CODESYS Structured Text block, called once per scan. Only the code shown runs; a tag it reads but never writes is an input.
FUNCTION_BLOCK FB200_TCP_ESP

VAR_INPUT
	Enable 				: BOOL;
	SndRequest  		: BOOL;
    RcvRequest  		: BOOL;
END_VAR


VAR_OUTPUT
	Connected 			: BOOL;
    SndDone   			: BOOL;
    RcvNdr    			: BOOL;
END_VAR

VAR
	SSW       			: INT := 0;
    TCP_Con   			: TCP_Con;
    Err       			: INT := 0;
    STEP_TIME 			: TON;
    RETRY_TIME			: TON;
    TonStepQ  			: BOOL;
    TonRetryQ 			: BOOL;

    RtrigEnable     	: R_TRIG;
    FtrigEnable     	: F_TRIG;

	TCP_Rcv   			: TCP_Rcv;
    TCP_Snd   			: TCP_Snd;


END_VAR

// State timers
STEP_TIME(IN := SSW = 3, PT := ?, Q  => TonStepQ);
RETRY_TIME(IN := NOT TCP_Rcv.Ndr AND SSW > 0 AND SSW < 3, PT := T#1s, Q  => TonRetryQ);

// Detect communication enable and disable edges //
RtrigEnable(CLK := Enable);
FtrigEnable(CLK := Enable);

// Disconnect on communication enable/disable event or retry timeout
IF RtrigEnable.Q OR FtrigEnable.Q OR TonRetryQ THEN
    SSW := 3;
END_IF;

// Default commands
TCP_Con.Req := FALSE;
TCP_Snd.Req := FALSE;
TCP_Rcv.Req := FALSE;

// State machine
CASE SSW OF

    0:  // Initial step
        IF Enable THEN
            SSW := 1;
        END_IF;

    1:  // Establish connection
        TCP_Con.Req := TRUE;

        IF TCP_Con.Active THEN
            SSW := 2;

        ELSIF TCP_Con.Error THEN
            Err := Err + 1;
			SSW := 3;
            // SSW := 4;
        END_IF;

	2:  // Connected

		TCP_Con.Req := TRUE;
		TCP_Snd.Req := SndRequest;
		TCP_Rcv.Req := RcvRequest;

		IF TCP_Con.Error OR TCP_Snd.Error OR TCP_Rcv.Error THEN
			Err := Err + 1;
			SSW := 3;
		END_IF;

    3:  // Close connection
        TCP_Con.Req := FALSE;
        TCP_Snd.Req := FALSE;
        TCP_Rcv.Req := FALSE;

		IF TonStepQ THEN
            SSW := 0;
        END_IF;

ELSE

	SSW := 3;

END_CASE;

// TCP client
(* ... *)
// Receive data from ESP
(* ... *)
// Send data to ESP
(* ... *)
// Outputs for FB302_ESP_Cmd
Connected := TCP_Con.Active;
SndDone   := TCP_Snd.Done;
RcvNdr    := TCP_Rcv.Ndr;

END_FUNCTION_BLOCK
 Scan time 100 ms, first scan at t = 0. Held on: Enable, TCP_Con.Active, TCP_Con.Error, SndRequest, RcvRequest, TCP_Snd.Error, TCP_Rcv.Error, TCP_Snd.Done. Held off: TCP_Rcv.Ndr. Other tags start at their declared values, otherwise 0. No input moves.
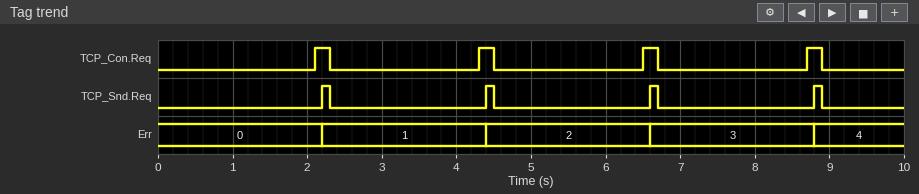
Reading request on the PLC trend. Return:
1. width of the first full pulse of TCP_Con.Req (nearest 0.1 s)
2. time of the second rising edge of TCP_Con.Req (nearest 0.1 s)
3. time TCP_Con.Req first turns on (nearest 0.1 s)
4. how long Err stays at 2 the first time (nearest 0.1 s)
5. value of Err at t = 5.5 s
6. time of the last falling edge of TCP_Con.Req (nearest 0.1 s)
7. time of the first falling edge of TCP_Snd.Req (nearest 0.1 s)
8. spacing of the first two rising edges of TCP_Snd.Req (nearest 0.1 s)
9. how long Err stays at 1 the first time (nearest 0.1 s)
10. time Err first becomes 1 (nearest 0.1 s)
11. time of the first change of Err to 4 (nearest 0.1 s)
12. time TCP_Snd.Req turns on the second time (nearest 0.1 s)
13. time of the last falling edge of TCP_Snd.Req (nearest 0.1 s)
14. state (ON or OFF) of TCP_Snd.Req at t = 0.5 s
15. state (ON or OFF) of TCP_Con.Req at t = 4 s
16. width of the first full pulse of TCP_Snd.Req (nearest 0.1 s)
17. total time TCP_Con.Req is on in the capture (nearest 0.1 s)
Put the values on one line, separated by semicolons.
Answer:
0.2 s; 4.3 s; 2.1 s; 2.2 s; 2; 8.9 s; 2.3 s; 2.2 s; 2.2 s; 2.2 s; 8.8 s; 4.4 s; 8.9 s; OFF; OFF; 0.1 s; 0.8 s
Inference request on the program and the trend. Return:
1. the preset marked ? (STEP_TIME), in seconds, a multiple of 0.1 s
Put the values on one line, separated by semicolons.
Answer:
1.8 s
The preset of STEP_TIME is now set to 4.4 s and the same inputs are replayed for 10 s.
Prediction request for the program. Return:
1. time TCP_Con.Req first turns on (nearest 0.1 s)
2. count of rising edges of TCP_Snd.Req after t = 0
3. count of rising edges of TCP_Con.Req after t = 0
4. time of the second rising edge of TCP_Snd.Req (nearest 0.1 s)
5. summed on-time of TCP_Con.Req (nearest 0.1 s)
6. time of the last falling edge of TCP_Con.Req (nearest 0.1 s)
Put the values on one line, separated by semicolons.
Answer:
4.7 s; 2; 2; 9.6 s; 0.4 s; 9.7 s
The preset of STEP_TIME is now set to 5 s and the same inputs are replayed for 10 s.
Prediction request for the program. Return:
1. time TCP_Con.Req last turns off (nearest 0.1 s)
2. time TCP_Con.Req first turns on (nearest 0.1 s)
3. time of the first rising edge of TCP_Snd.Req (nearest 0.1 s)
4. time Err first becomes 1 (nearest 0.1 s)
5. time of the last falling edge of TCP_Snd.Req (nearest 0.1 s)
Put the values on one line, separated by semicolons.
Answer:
5.5 s; 5.3 s; 5.4 s; 5.4 s; 5.5 s
